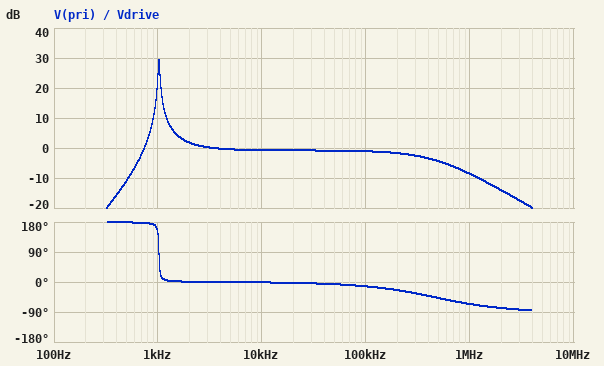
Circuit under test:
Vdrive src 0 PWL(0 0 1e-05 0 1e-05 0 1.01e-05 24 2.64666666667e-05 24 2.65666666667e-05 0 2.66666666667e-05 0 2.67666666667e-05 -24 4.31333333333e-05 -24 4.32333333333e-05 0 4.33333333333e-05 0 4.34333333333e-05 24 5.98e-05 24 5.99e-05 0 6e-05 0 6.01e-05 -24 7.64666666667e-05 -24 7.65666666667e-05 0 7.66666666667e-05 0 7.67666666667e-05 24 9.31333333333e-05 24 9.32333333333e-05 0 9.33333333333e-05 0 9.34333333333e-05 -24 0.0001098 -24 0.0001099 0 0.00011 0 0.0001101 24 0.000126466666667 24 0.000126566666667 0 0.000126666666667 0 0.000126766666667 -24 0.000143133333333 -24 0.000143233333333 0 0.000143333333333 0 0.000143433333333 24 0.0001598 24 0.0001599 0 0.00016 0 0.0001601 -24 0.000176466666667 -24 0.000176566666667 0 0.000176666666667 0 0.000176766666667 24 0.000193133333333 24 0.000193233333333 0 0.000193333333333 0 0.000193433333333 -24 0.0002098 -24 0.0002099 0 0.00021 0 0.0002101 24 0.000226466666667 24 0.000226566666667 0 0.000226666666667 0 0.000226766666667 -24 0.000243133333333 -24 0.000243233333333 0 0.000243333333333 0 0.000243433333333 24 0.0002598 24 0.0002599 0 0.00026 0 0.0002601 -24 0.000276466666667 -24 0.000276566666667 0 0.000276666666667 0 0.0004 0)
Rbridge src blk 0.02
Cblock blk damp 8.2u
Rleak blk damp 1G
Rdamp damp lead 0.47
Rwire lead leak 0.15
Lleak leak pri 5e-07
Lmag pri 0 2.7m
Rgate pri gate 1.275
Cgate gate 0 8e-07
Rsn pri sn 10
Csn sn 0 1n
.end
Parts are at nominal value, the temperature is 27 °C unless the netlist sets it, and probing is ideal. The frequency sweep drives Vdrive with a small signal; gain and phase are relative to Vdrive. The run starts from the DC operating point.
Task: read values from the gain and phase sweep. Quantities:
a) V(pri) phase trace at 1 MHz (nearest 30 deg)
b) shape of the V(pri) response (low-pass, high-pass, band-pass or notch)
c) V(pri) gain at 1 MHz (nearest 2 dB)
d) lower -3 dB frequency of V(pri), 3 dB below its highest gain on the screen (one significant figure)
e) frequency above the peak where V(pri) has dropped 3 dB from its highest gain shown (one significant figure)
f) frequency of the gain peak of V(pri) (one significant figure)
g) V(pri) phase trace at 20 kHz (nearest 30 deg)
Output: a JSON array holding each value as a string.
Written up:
["-60 deg", "band-pass", "-8 dB", "1 kHz", "1 kHz", "1 kHz", "0 deg"]
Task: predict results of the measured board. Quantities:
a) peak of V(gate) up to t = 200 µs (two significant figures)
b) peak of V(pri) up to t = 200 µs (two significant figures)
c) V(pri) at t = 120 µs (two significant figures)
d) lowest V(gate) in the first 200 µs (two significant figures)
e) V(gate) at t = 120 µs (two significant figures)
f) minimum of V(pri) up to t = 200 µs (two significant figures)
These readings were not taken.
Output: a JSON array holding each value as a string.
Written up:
["22 V", "22 V", "21 V", "-23 V", "21 V", "-23 V"]
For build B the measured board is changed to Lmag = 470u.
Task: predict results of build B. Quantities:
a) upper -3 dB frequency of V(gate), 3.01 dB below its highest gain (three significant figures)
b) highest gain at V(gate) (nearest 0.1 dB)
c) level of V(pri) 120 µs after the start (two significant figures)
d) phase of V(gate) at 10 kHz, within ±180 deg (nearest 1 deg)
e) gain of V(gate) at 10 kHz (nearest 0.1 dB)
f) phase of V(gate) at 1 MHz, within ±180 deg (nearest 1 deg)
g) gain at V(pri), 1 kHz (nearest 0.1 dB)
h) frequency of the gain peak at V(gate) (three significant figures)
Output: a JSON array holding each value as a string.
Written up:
["2.55 kHz", "21.7 dB", "19 V", "-4 deg", "-0.3 dB", "-147 deg", "-14.8 dB", "2.45 kHz"]
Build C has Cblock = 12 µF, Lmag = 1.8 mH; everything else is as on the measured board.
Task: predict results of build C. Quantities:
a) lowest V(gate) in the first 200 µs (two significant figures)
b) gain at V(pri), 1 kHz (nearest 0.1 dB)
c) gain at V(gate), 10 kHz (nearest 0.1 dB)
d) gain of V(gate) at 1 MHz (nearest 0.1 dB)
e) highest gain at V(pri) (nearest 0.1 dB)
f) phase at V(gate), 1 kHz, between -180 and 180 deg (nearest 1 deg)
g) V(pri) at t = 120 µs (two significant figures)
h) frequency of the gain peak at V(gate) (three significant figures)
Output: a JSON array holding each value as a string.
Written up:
["-24 V", "18.5 dB", "-0.5 dB", "-24.9 dB", "25.8 dB", "153 deg", "22 V", "1.05 kHz"]
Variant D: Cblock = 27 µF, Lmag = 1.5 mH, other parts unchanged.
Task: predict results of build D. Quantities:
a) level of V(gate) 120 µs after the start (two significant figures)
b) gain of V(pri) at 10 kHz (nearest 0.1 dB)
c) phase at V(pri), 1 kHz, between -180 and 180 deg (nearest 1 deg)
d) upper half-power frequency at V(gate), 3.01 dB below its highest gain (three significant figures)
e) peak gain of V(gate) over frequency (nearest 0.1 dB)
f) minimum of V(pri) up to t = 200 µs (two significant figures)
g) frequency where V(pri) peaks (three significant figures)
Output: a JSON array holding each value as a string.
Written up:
["23 V", "-0.2 dB", "9 deg", "815 Hz", "21.4 dB", "-24 V", "781 Hz"]
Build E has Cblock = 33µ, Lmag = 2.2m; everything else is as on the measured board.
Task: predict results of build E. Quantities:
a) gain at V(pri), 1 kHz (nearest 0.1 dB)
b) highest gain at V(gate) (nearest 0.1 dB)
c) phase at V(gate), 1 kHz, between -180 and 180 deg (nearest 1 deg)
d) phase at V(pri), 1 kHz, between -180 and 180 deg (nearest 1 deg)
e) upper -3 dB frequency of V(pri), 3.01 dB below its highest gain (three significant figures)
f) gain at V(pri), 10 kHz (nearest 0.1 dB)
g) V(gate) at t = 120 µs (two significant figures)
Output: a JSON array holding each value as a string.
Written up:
["3.4 dB", "22.2 dB", "3 deg", "4 deg", "608 Hz", "-0.2 dB", "23 V"]
